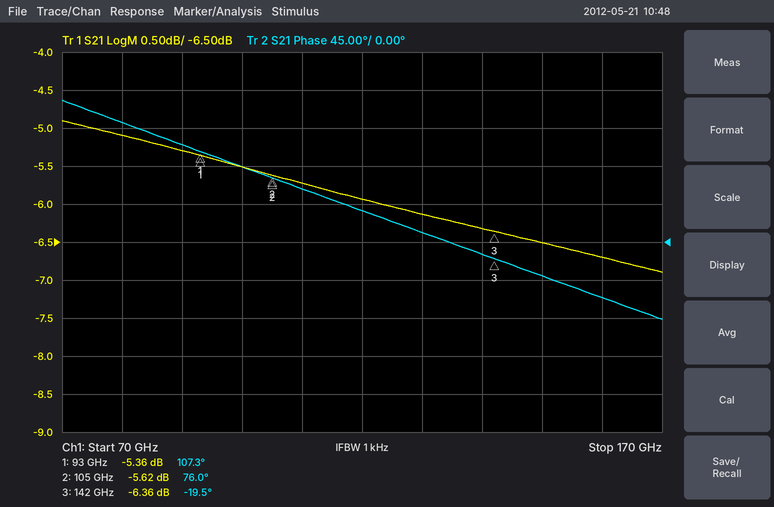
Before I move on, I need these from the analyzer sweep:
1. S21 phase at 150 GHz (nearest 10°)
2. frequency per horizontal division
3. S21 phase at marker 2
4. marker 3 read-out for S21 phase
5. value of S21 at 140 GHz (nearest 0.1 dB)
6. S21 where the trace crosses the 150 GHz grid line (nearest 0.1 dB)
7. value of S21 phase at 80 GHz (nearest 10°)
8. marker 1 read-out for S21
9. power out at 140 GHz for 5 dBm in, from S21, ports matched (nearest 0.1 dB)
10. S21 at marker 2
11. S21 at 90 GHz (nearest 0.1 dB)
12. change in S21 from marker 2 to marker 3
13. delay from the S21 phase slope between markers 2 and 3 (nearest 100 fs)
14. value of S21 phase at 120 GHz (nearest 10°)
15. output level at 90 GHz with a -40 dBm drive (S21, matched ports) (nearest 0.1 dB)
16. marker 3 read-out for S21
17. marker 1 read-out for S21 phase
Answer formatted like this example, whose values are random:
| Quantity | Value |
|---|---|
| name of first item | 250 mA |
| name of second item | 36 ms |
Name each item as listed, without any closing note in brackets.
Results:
| Quantity | Value |
|---|---|
| S21 phase at 150 GHz | -40° |
| frequency per horizontal division | 10 GHz |
| S21 phase at marker 2 | 76.0° |
| marker 3 read-out for S21 phase | -19.5° |
| value of S21 at 140 GHz | -6.3 dB |
| S21 where the trace crosses the 150 GHz grid line | -6.5 dB |
| value of S21 phase at 80 GHz | 140° |
| marker 1 read-out for S21 | -5.36 dB |
| power out at 140 GHz for 5 dBm in, from S21, ports matched | -1.3 dBm |
| S21 at marker 2 | -5.62 dB |
| S21 at 90 GHz | -5.3 dB |
| change in S21 from marker 2 to marker 3 | -0.74 dB |
| delay from the S21 phase slope between markers 2 and 3 | 7.2 ps |
| value of S21 phase at 120 GHz | 40° |
| output level at 90 GHz with a -40 dBm drive (S21, matched ports) | -45.3 dBm |
| marker 3 read-out for S21 | -6.36 dB |
| marker 1 read-out for S21 phase | 107.3° |
